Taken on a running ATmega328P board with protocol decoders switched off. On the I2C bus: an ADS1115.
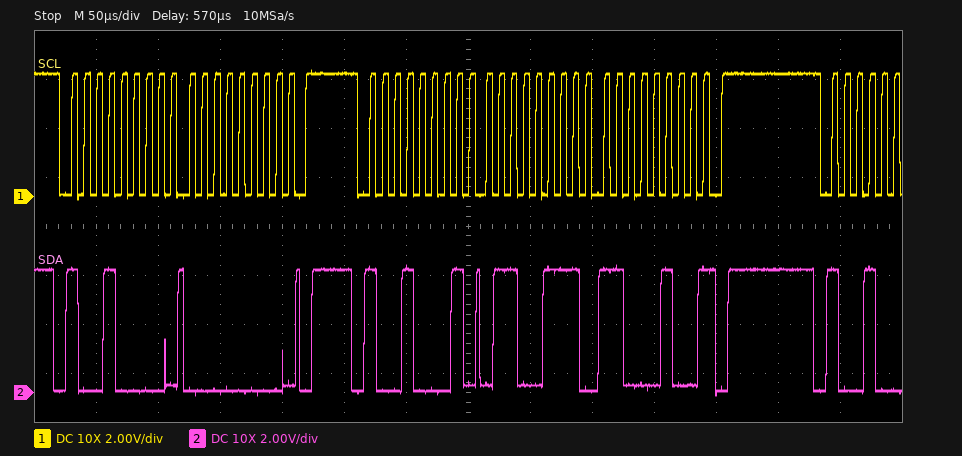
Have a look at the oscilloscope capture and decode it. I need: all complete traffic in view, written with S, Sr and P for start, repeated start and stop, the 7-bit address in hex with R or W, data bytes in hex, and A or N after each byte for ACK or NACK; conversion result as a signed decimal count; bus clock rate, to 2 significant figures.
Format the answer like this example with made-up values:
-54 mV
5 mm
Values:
S 48W A 00 A P S 48R A 67 A C4 N P
26564
100 kHz
